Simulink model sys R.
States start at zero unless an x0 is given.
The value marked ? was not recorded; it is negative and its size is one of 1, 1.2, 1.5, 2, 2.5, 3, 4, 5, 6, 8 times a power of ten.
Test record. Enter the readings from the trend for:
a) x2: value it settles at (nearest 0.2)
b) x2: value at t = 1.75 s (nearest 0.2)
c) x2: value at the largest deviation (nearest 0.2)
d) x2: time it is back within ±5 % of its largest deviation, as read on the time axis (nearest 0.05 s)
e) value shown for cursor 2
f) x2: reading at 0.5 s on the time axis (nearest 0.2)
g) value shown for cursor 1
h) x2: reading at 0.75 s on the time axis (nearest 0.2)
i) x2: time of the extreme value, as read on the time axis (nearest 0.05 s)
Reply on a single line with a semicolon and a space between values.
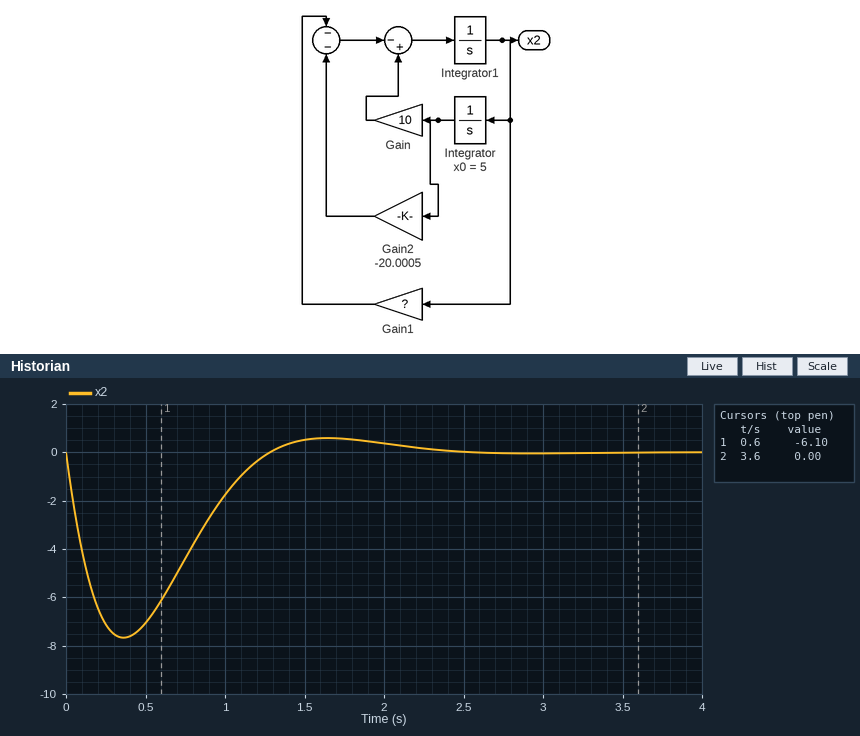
0.0; 0.6; -7.6; 2.00 s; 0.00; -7.0; -6.10; -4.4; 0.35 s
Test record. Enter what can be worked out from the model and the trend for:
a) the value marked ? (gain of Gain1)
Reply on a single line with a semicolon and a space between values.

-4
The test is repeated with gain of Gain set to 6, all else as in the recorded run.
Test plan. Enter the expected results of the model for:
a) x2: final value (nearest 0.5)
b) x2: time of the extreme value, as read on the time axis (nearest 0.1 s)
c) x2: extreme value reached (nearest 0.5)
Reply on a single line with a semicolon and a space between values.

0.0; 0.3 s; -10.0
